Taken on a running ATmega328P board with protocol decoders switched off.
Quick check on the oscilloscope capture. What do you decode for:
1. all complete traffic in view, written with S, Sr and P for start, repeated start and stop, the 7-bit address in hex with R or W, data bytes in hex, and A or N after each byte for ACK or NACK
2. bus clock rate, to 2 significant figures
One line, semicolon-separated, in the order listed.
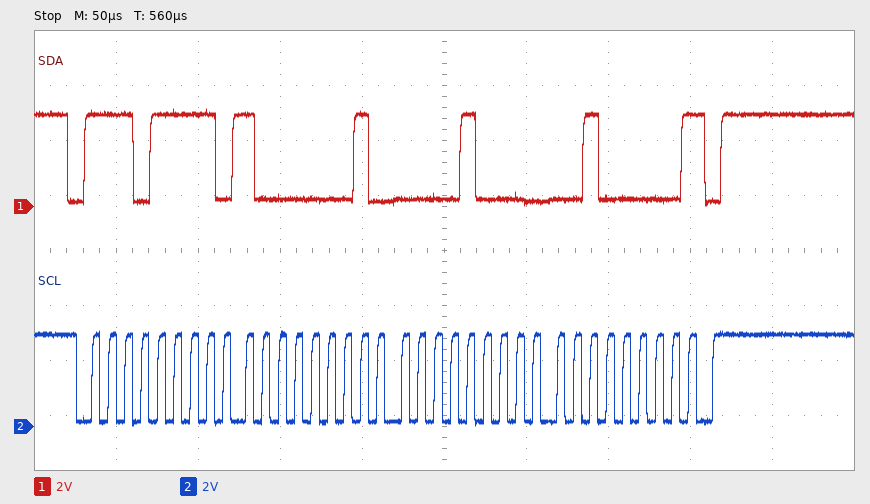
S 77R A 81 A 08 A 20 N P; 100 kHz
